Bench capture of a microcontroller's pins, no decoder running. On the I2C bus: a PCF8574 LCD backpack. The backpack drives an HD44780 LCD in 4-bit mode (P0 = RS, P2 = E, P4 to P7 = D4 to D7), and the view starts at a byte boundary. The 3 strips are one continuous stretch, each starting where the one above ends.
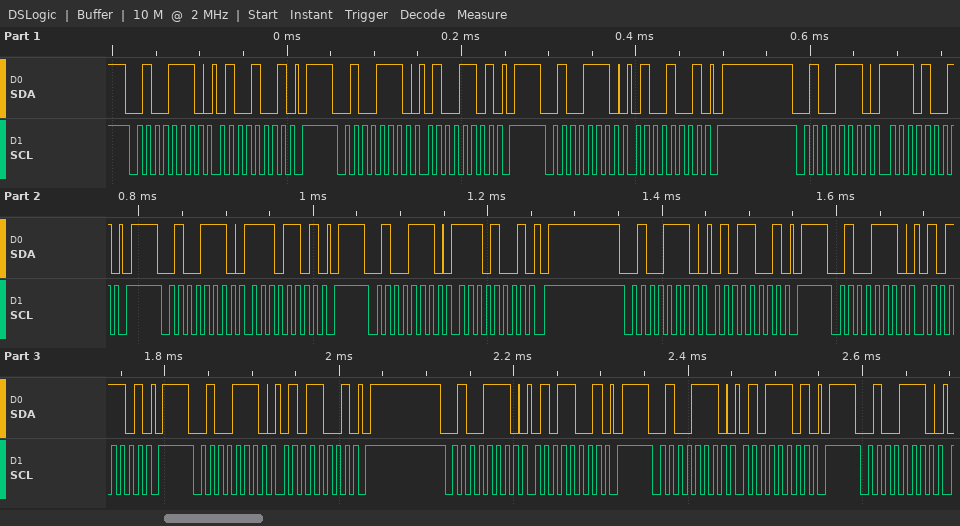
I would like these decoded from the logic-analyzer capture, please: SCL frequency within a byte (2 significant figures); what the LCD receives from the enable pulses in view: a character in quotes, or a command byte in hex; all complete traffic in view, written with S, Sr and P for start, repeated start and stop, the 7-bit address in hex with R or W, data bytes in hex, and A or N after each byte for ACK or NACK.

100 kHz
'N'
S 27W A 49 A P S 27W A 4D A P S 27W A 49 A P S 27W A E9 A P S 27W A ED A P S 27W A E9 A P S 27W A 59 A P S 27W A 5D A P S 27W A 59 A P S 27W A 59 A P S 27W A 5D A P S 27W A
